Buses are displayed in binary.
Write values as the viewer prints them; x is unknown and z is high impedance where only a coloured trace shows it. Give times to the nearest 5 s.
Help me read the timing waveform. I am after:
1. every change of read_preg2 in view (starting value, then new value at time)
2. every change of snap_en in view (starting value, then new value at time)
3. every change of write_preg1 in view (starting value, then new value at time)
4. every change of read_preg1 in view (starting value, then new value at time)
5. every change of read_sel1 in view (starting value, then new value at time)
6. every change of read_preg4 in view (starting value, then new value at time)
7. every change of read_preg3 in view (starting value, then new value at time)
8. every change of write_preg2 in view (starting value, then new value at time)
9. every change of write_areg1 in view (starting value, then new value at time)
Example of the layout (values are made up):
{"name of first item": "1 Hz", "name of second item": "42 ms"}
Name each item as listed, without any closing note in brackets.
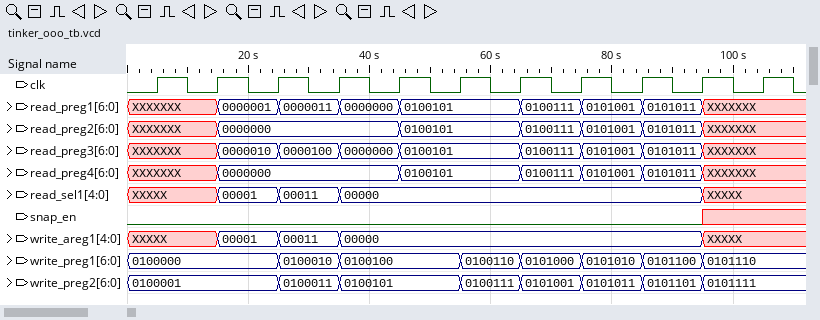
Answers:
{"every change of read_preg2 in view": "XXXXXXX, 0000000 at 15 s, 0100101 at 45 s, 0100111 at 65 s, 0101001 at 75 s, 0101011 at 85 s, XXXXXXX at 95 s", "every change of snap_en in view": "0, x at 95 s", "every change of write_preg1 in view": "0100000, 0100010 at 25 s, 0100100 at 35 s, 0100110 at 55 s, 0101000 at 65 s, 0101010 at 75 s, 0101100 at 85 s, 0101110 at 95 s", "every change of read_preg1 in view": "XXXXXXX, 0000001 at 15 s, 0000011 at 25 s, 0000000 at 35 s, 0100101 at 45 s, 0100111 at 65 s, 0101001 at 75 s, 0101011 at 85 s, XXXXXXX at 95 s", "every change of read_sel1 in view": "XXXXX, 00001 at 15 s, 00011 at 25 s, 00000 at 35 s, XXXXX at 95 s", "every change of read_preg4 in view": "XXXXXXX, 0000000 at 15 s, 0100101 at 45 s, 0100111 at 65 s, 0101001 at 75 s, 0101011 at 85 s, XXXXXXX at 95 s", "every change of read_preg3 in view": "XXXXXXX, 0000010 at 15 s, 0000100 at 25 s, 0000000 at 35 s, 0100101 at 45 s, 0100111 at 65 s, 0101001 at 75 s, 0101011 at 85 s, XXXXXXX at 95 s", "every change of write_preg2 in view": "0100001, 0100011 at 25 s, 0100101 at 35 s, 0100111 at 55 s, 0101001 at 65 s, 0101011 at 75 s, 0101101 at 85 s, 0101111 at 95 s", "every change of write_areg1 in view": "XXXXX, 00001 at 15 s, 00011 at 25 s, 00000 at 35 s, XXXXX at 95 s"}
